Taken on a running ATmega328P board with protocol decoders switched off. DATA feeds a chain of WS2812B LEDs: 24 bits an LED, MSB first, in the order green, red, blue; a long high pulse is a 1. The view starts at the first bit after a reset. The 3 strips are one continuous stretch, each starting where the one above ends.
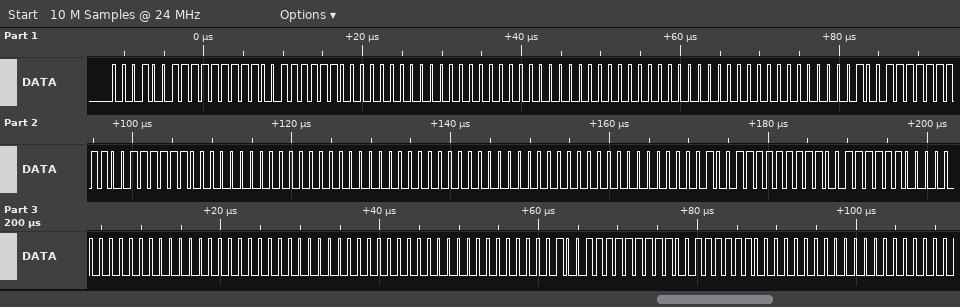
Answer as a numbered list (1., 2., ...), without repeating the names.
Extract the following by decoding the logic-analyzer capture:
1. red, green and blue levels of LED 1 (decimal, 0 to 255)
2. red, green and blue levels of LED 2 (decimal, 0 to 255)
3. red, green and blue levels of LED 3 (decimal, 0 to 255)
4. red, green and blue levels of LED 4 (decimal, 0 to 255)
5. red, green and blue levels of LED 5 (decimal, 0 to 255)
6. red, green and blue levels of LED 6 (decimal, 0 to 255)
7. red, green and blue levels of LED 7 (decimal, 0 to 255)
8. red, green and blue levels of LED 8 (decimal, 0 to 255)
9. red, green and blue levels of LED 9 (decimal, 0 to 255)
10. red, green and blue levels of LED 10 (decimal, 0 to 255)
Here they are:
1. 254, 19, 126
2. 0, 0, 0
3. 0, 0, 0
4. 254, 19, 126
5. 0, 0, 0
6. 0, 0, 0
7. 254, 19, 126
8. 0, 0, 0
9. 0, 0, 0
10. 254, 19, 126
